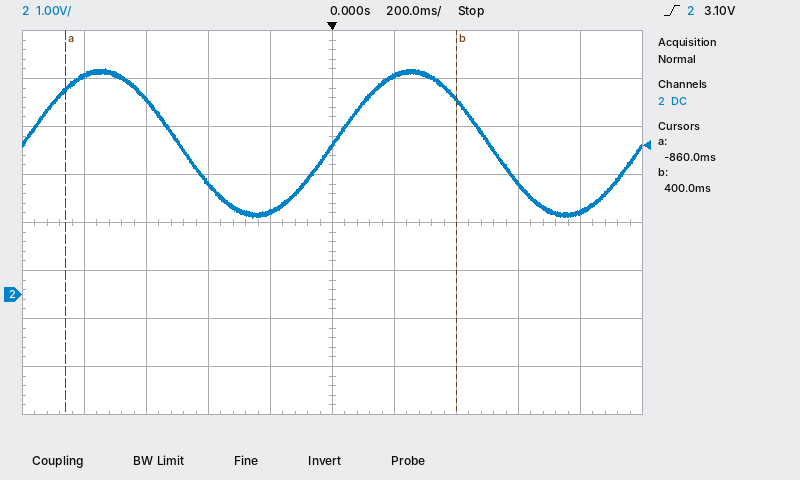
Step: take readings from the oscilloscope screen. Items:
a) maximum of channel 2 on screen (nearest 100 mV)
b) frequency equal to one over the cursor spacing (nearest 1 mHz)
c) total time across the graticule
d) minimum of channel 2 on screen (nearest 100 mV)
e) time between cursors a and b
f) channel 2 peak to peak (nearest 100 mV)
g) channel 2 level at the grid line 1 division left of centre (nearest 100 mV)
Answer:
4.7 V
794 mHz
2 s
1.6 V
1.26 s
3.1 V
1.7 V
